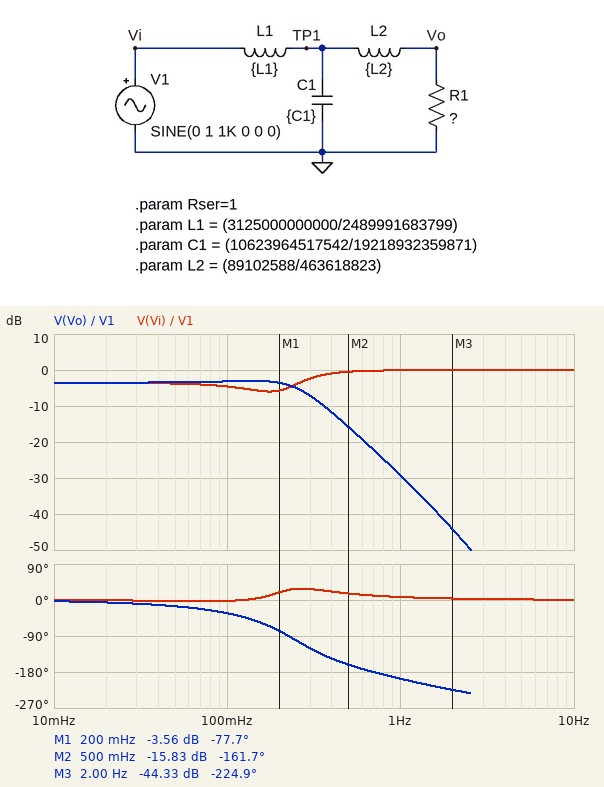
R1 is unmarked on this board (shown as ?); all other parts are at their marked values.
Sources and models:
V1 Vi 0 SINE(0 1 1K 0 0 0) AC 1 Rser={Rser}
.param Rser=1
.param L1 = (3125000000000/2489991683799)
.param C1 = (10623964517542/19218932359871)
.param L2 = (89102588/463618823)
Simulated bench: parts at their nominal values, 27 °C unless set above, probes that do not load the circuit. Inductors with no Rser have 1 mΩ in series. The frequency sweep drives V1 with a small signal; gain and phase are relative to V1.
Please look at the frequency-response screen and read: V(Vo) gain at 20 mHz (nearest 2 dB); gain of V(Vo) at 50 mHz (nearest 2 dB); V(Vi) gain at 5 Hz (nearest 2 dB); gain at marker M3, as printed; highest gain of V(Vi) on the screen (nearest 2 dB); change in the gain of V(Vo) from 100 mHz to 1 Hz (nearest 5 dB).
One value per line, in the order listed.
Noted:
-4 dB
-4 dB
0 dB
-44.33 dB
0 dB
-25 dB
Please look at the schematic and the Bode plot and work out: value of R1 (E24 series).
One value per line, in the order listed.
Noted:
2 Ω
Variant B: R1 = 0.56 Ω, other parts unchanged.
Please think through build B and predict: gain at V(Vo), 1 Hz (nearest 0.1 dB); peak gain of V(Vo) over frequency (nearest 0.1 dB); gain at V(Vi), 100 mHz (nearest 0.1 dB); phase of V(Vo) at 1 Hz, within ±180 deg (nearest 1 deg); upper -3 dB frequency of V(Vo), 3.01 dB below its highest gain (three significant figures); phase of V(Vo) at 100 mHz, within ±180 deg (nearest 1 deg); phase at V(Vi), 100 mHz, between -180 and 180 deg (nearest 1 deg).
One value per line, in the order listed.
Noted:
-34.1 dB
-8.9 dB
-5.1 dB
129 deg
232 mHz
-38 deg
27 deg
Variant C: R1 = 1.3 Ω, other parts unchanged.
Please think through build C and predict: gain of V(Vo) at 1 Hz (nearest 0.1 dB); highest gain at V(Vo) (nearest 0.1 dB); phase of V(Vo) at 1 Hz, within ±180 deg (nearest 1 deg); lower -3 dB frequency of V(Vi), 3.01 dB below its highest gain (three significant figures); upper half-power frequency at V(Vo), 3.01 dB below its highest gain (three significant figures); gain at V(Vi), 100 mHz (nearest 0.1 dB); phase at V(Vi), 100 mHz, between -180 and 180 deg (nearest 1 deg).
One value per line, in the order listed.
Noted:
-30.2 dB
-5.0 dB
153 deg
262 mHz
285 mHz
-5.1 dB
8 deg
